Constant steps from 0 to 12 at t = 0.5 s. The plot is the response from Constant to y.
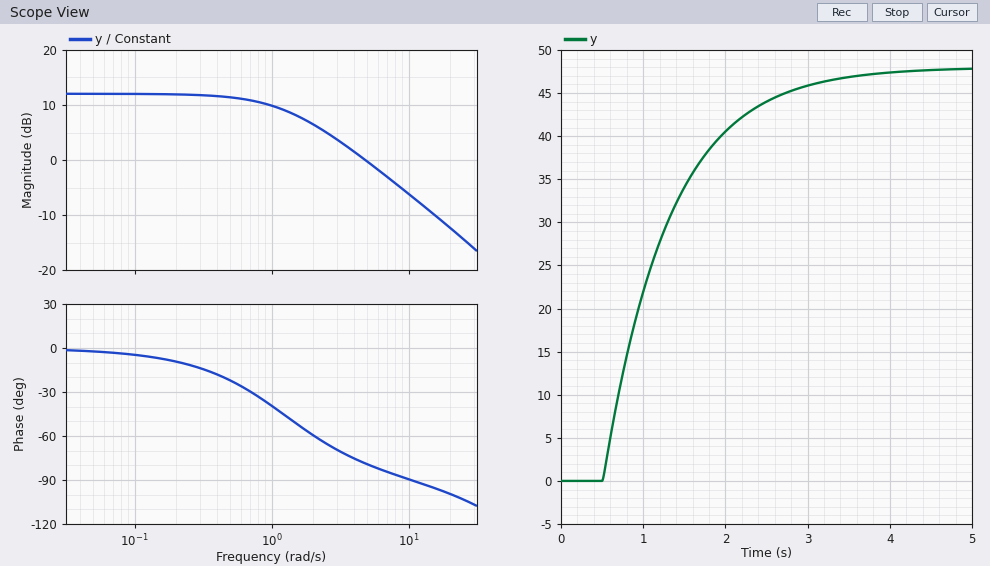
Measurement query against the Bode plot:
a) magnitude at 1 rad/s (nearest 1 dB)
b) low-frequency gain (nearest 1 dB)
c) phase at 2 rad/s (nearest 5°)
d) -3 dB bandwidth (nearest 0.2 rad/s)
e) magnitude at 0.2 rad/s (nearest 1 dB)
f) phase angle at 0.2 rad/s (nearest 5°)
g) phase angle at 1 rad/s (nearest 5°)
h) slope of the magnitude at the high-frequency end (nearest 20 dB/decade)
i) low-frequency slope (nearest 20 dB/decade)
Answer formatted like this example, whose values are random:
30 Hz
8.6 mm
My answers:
10 dB
12 dB
-60°
1.2 rad/s
12 dB
-10°
-40°
-20 dB/decade
0 dB/decade
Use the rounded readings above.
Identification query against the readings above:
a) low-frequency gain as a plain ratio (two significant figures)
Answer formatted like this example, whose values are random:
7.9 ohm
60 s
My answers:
4.0
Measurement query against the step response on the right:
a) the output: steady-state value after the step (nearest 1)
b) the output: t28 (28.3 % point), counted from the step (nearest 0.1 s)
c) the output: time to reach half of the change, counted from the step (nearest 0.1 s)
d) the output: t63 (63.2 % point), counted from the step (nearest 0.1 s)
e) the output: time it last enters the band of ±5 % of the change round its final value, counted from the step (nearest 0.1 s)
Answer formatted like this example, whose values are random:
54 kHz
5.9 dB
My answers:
48
0.3 s
0.6 s
0.8 s
2.4 s
